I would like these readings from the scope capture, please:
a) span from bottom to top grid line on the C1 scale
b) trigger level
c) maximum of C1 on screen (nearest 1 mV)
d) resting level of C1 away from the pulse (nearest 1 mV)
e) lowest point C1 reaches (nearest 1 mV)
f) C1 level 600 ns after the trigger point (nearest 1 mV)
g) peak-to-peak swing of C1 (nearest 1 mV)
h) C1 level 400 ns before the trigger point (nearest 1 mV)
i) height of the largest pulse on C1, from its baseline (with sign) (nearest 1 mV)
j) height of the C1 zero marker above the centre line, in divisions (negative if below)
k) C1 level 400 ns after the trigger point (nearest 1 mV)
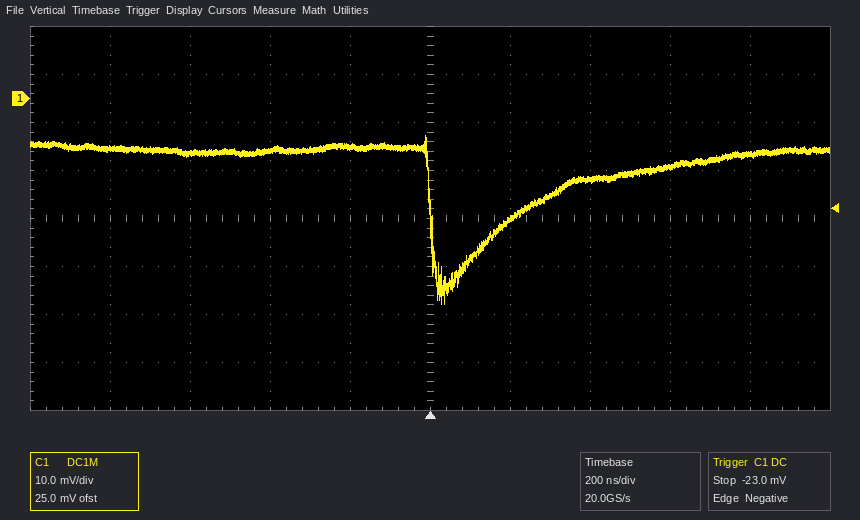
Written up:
80 mV
-23.0 mV
-8 mV
-11 mV
-43 mV
-14 mV
35 mV
-11 mV
-32 mV
+2.5 div
-17 mV
